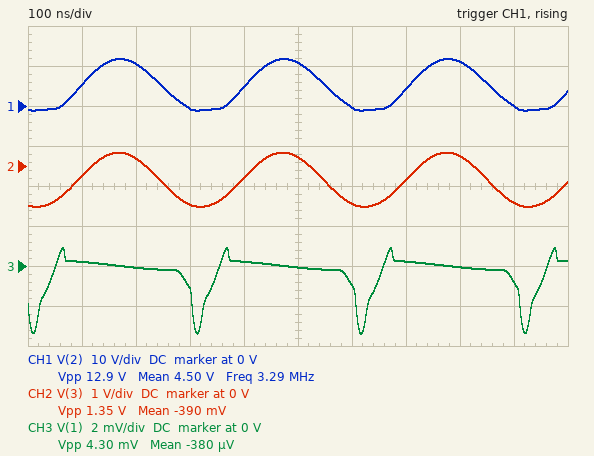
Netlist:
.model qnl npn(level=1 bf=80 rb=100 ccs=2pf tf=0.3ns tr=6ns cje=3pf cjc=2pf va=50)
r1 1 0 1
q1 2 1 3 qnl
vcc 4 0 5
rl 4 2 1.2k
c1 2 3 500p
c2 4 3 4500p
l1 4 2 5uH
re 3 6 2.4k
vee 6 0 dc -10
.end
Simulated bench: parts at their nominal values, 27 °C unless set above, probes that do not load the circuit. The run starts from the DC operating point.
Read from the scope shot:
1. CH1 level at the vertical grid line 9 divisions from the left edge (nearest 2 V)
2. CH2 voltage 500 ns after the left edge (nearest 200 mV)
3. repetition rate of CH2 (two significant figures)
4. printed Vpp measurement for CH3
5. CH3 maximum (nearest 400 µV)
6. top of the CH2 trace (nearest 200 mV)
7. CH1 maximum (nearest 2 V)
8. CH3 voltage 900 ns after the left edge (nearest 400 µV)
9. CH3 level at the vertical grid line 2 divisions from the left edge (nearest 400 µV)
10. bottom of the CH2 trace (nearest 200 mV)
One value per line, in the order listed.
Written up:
0 V
200 mV
3.3 MHz
4.30 mV
800 µV
400 mV
12 V
-800 µV
0 V
-1.0 V
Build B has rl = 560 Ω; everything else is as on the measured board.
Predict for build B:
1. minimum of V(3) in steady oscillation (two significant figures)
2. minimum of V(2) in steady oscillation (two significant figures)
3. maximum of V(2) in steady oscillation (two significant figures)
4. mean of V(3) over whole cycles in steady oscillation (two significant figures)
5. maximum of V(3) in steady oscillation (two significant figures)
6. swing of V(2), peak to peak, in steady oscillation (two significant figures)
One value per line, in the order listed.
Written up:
-900 mV
1.1 V
8.7 V
-530 mV
-150 mV
7.6 V
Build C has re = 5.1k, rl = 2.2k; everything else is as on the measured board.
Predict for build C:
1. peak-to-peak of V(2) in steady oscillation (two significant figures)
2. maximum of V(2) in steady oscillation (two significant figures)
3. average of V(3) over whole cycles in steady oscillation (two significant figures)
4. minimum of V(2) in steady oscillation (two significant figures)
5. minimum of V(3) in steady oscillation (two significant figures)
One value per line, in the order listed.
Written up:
12 V
11 V
-300 mV
-970 mV
-930 mV
